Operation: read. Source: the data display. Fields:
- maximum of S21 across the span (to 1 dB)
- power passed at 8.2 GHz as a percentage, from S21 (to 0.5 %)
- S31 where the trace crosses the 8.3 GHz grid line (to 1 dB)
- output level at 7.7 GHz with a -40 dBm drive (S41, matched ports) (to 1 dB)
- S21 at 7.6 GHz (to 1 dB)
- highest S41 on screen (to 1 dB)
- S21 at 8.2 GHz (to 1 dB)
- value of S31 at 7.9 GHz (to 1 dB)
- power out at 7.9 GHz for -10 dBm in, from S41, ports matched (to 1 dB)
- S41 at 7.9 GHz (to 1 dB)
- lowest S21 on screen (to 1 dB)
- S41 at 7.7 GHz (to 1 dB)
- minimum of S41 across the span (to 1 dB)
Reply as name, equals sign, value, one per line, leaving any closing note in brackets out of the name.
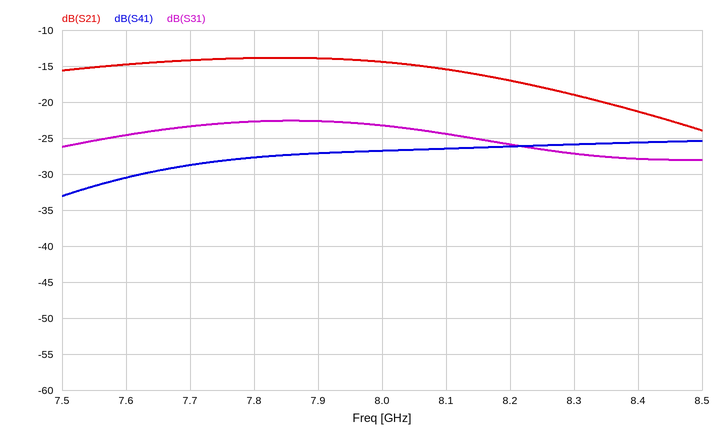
maximum of S21 across the span = -14 dB
power passed at 8.2 GHz as a percentage, from S21 = 2.0 %
S31 where the trace crosses the 8.3 GHz grid line = -27 dB
output level at 7.7 GHz with a -40 dBm drive (S41, matched ports) = -69 dBm
S21 at 7.6 GHz = -15 dB
highest S41 on screen = -25 dB
S21 at 8.2 GHz = -17 dB
value of S31 at 7.9 GHz = -23 dB
power out at 7.9 GHz for -10 dBm in, from S41, ports matched = -37 dBm
S41 at 7.9 GHz = -27 dB
lowest S21 on screen = -24 dB
S41 at 7.7 GHz = -29 dB
minimum of S41 across the span = -33 dB
